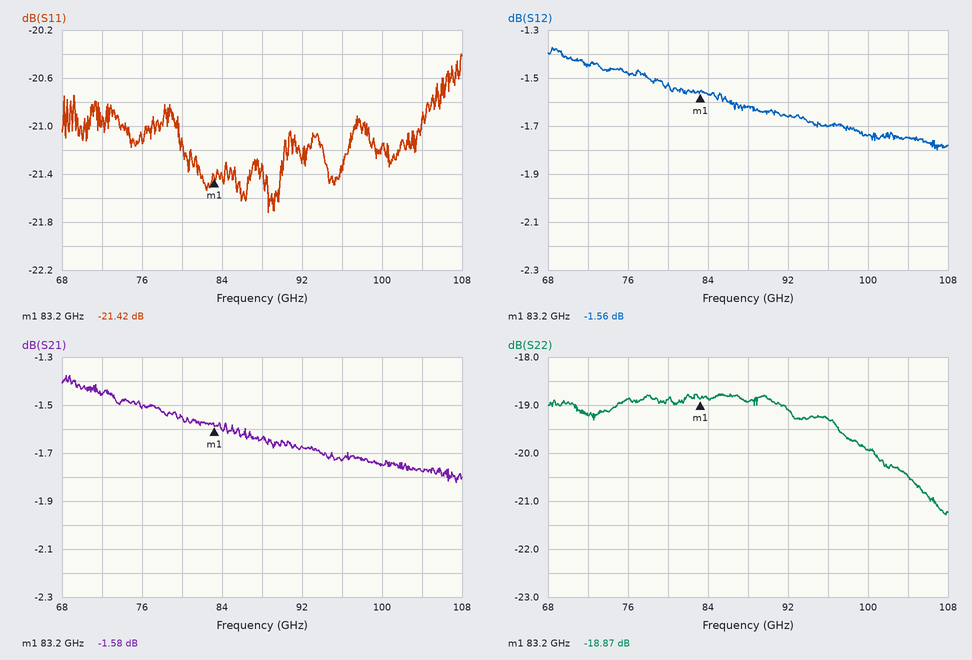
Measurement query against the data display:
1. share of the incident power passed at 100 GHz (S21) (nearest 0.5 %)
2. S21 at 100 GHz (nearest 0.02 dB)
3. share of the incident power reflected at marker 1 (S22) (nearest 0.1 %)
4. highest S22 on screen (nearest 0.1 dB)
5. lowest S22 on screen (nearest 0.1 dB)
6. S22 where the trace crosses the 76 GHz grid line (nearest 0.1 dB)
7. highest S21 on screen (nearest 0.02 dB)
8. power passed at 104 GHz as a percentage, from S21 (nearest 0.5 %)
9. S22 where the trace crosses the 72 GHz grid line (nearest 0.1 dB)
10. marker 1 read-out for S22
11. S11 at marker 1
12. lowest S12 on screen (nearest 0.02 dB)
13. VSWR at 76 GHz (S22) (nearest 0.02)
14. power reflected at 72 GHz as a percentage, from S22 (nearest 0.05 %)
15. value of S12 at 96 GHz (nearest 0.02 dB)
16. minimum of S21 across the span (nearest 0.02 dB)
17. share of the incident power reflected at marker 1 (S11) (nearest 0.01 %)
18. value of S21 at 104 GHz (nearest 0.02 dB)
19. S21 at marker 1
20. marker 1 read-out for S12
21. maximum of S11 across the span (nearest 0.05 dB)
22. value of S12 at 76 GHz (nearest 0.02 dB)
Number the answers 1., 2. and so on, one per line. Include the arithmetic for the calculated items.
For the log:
1. 10^(-1.74/10) ≈ 67.0 %
2. -1.74 dB
3. 10^(-18.87/10) ≈ 1.3 %
4. -18.8 dB
5. -21.3 dB
6. -18.9 dB
7. -1.38 dB
8. 10^(-1.78/10) ≈ 66.4 %, so 66.5 % to the nearest 0.5 %
9. -19.2 dB
10. -18.87 dB
11. -21.42 dB
12. -1.80 dB
13. |Γ| = 10^(-18.9/20) = 0.1135; VSWR = (1 + 0.1135)/(1 − 0.1135) ≈ 1.26
14. 10^(-19.2/10) ≈ 1.20 %
15. -1.70 dB
16. -1.82 dB
17. 10^(-21.42/10) ≈ 0.72 %
18. -1.78 dB
19. -1.58 dB
20. -1.56 dB
21. -20.40 dB
22. -1.48 dB
